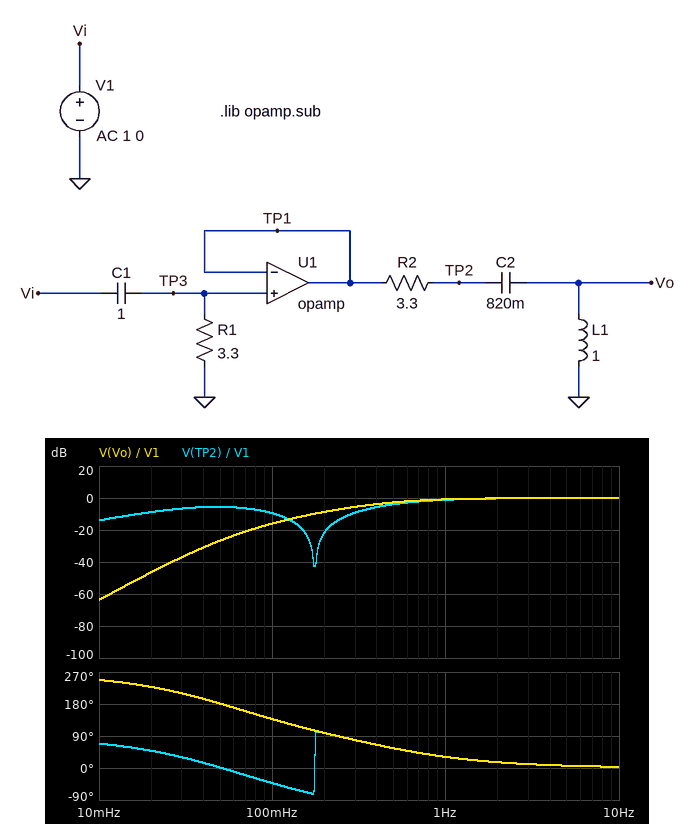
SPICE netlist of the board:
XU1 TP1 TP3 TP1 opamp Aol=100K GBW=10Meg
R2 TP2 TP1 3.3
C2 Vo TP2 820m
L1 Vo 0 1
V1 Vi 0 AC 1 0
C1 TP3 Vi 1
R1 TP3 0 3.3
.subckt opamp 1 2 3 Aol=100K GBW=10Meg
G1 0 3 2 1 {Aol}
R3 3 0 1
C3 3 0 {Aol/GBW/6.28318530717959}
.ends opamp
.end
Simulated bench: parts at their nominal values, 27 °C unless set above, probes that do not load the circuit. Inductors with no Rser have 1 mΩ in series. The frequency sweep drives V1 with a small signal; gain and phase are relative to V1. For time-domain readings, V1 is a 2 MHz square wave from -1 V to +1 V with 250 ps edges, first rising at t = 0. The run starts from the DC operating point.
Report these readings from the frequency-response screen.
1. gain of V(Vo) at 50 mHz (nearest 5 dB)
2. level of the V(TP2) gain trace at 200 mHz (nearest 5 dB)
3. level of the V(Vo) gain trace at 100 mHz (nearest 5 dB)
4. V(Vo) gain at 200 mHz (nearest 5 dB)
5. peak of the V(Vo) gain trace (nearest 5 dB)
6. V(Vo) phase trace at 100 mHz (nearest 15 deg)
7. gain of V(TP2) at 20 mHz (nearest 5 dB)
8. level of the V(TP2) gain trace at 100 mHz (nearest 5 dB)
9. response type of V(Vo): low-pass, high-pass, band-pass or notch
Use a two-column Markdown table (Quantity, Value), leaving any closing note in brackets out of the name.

| Quantity | Value |
|---|---|
| gain of V(Vo) at 50 mHz | -25 dB |
| level of the V(TP2) gain trace at 200 mHz | -20 dB |
| level of the V(Vo) gain trace at 100 mHz | -15 dB |
| V(Vo) gain at 200 mHz | -10 dB |
| peak of the V(Vo) gain trace | 0 dB |
| V(Vo) phase trace at 100 mHz | 135 deg |
| gain of V(TP2) at 20 mHz | -10 dB |
| level of the V(TP2) gain trace at 100 mHz | -10 dB |
| response type of V(Vo): low-pass, high-pass, band-pass or notch | high-pass |
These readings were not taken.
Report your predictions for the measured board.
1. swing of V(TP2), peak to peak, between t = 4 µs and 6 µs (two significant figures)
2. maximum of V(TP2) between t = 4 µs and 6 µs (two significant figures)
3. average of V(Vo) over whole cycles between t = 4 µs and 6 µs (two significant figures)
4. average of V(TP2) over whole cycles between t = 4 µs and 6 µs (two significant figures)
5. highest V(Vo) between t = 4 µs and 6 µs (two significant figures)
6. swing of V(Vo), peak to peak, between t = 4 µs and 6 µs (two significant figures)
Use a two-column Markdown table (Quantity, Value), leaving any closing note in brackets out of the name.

| Quantity | Value |
|---|---|
| swing of V(TP2), peak to peak, between t = 4 µs and 6 µs | 2.0 V |
| maximum of V(TP2) between t = 4 µs and 6 µs | 2.0 V |
| average of V(Vo) over whole cycles between t = 4 µs and 6 µs | 1.0 V |
| average of V(TP2) over whole cycles between t = 4 µs and 6 µs | 1.0 V |
| highest V(Vo) between t = 4 µs and 6 µs | 2.0 V |
| swing of V(Vo), peak to peak, between t = 4 µs and 6 µs | 2.0 V |
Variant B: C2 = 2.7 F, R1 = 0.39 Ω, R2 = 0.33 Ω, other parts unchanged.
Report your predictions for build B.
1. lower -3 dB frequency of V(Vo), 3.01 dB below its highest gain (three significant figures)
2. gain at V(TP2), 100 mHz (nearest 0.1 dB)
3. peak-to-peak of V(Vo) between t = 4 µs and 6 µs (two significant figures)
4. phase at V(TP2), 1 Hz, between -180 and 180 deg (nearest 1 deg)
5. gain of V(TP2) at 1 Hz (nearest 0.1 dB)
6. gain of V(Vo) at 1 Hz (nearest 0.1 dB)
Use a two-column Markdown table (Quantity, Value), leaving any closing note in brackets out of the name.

| Quantity | Value |
|---|---|
| lower -3 dB frequency of V(Vo), 3.01 dB below its highest gain | 363 mHz |
| gain at V(TP2), 100 mHz | -31.1 dB |
| peak-to-peak of V(Vo) between t = 4 µs and 6 µs | 2.0 V |
| phase at V(TP2), 1 Hz, between -180 and 180 deg | 25 deg |
| gain of V(TP2) at 1 Hz | -0.7 dB |
| gain of V(Vo) at 1 Hz | -0.6 dB |
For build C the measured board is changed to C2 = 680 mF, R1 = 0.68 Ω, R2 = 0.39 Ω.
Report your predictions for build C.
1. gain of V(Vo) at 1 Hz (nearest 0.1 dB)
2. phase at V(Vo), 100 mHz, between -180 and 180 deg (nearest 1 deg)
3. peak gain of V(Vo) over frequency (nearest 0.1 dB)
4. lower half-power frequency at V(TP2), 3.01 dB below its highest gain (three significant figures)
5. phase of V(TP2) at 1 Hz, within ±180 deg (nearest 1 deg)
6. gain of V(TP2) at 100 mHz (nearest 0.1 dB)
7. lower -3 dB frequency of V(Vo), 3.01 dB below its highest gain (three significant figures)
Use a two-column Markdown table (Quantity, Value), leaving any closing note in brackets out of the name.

| Quantity | Value |
|---|---|
| gain of V(Vo) at 1 Hz | 0.1 dB |
| phase at V(Vo), 100 mHz, between -180 and 180 deg | -126 deg |
| peak gain of V(Vo) over frequency | 6.2 dB |
| lower half-power frequency at V(TP2), 3.01 dB below its highest gain | 280 mHz |
| phase of V(TP2) at 1 Hz, within ±180 deg | 17 deg |
| gain of V(TP2) at 100 mHz | -8.3 dB |
| lower -3 dB frequency of V(Vo), 3.01 dB below its highest gain | 175 mHz |
